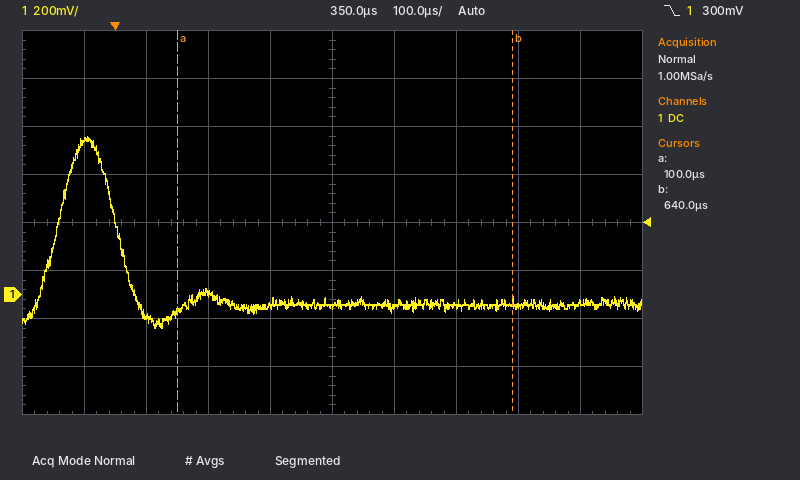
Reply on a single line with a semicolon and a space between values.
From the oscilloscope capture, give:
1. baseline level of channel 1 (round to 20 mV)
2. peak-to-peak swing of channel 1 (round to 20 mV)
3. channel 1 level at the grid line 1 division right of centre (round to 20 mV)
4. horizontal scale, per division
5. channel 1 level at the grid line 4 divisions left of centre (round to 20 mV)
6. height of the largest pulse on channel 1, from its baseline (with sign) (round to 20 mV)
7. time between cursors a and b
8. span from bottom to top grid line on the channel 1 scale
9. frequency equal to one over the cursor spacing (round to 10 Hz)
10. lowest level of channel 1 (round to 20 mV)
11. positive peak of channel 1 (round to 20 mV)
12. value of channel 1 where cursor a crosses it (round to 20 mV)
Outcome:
-40 mV; 800 mV; -60 mV; 100 µs; 640 mV; +700 mV; 540 µs; 1.6 V; 1.85 kHz; -140 mV; 660 mV; -80 mV
